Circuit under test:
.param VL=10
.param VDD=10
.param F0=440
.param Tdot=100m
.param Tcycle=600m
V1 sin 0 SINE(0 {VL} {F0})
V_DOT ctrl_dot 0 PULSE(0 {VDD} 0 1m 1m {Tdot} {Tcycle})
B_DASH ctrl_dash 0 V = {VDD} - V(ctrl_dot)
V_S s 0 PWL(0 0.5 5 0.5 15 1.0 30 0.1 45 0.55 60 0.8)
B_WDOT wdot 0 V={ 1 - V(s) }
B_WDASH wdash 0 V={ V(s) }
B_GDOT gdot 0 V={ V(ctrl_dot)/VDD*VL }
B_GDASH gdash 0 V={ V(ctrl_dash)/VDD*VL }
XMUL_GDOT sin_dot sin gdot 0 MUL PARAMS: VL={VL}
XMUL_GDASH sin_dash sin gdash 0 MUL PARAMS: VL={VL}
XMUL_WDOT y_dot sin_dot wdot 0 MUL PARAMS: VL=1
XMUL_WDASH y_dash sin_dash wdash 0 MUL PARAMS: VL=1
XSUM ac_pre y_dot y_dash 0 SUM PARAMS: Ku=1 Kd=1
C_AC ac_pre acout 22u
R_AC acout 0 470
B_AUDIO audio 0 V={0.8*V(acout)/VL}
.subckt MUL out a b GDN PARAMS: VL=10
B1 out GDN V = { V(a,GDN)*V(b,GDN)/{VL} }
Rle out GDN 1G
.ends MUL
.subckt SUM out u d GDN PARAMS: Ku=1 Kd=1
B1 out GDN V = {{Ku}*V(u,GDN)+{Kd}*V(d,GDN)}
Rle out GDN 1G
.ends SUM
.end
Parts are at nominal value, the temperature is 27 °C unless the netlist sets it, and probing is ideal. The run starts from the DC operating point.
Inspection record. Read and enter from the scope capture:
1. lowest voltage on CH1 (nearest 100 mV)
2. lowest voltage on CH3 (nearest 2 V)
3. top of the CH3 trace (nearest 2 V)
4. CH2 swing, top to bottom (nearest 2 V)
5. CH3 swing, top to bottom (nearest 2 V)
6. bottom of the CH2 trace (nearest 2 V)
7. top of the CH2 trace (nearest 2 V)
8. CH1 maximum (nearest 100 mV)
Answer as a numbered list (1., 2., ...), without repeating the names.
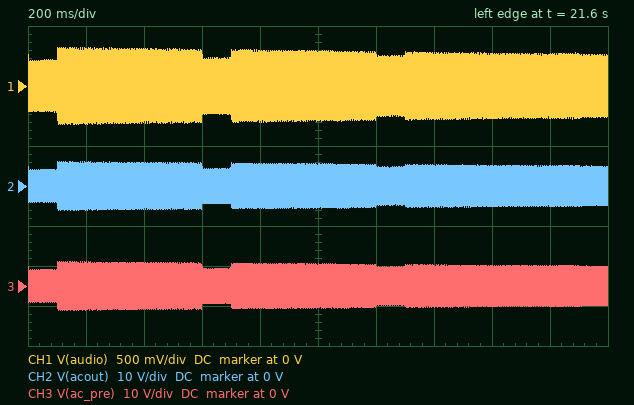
1. -500 mV
2. -6 V
3. 6 V
4. 12 V
5. 12 V
6. -6 V
7. 6 V
8. 500 mV
